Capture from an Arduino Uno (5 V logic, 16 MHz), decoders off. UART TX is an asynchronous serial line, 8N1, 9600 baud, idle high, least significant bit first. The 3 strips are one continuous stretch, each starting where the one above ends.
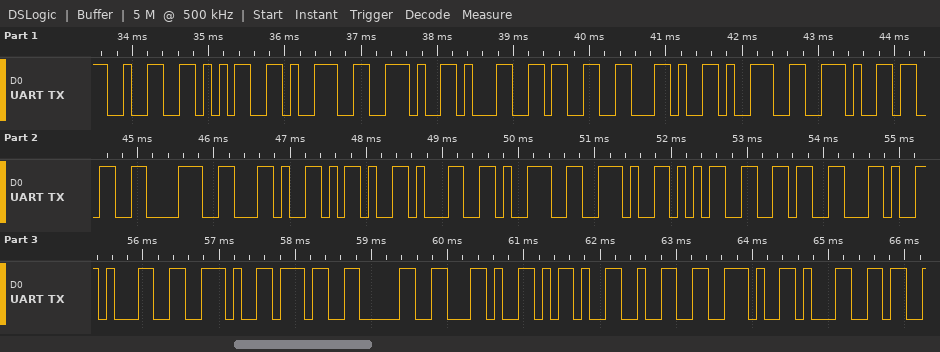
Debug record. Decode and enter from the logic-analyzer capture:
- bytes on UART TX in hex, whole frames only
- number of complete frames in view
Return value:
32 35 39 2E 31 33 2C 39 2E 33 38 2C 2D 31 39 2E 35 36 2C 31 2E 37 30 2C 2D 32 2E 31
28
